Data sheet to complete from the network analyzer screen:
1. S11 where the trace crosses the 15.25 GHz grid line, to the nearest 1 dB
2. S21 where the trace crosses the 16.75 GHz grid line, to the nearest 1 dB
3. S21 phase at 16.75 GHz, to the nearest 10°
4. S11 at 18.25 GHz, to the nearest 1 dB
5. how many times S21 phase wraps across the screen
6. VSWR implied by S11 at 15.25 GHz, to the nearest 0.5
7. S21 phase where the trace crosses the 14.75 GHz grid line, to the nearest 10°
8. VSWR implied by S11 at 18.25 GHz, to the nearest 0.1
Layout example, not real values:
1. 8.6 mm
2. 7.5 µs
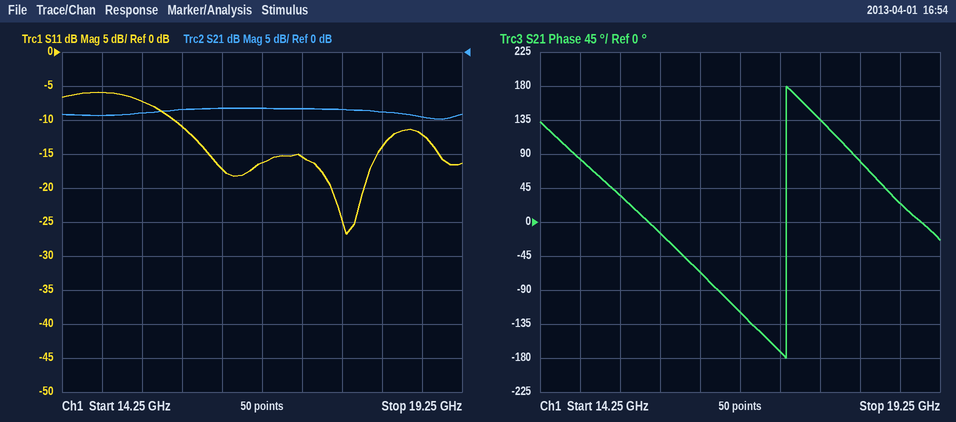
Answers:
1. -7 dB
2. -8 dB
3. -120°
4. -14 dB
5. 1
6. 2.5
7. 80°
8. 1.5
